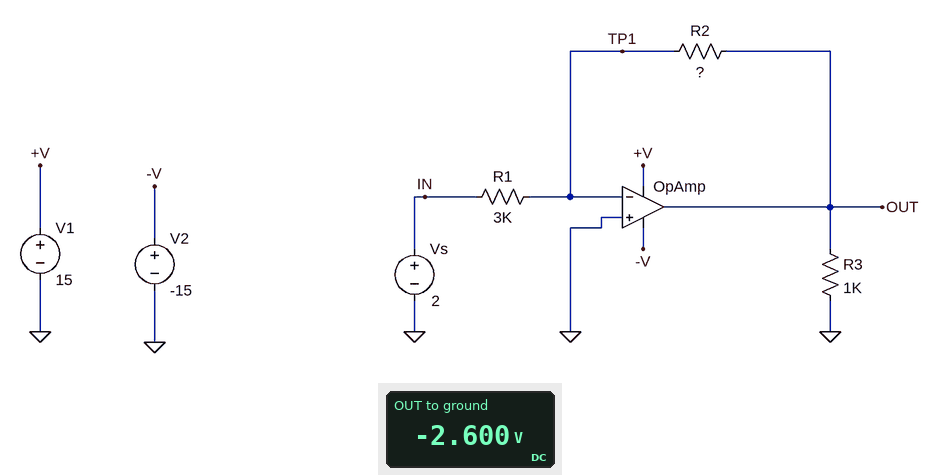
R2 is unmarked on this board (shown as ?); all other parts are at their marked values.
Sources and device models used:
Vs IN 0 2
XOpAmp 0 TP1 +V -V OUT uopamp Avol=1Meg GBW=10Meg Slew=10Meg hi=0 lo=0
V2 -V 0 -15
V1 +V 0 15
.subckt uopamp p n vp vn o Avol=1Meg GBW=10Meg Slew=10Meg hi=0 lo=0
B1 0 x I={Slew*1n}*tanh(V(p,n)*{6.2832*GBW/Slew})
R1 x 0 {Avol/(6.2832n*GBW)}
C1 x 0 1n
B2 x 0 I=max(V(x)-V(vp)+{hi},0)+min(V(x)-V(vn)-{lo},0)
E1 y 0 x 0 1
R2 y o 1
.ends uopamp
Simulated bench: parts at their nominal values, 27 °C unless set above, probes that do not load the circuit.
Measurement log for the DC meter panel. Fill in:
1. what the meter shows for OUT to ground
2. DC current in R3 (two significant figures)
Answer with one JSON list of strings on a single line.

["-2.600 V", "2.6 mA"]
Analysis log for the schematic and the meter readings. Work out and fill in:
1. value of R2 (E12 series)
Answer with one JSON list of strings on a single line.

["3.9 kΩ"]
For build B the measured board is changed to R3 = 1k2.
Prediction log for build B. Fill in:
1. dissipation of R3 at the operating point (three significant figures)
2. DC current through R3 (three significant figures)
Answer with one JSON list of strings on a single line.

["5.63 mW", "2.17 mA"]
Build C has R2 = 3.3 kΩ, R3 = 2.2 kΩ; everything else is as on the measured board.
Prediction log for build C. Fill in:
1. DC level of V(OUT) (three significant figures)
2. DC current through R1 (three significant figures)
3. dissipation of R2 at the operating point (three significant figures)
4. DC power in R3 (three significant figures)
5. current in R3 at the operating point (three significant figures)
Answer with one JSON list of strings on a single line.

["-2.20 V", "667 µA", "1.47 mW", "2.20 mW", "1.00 mA"]
